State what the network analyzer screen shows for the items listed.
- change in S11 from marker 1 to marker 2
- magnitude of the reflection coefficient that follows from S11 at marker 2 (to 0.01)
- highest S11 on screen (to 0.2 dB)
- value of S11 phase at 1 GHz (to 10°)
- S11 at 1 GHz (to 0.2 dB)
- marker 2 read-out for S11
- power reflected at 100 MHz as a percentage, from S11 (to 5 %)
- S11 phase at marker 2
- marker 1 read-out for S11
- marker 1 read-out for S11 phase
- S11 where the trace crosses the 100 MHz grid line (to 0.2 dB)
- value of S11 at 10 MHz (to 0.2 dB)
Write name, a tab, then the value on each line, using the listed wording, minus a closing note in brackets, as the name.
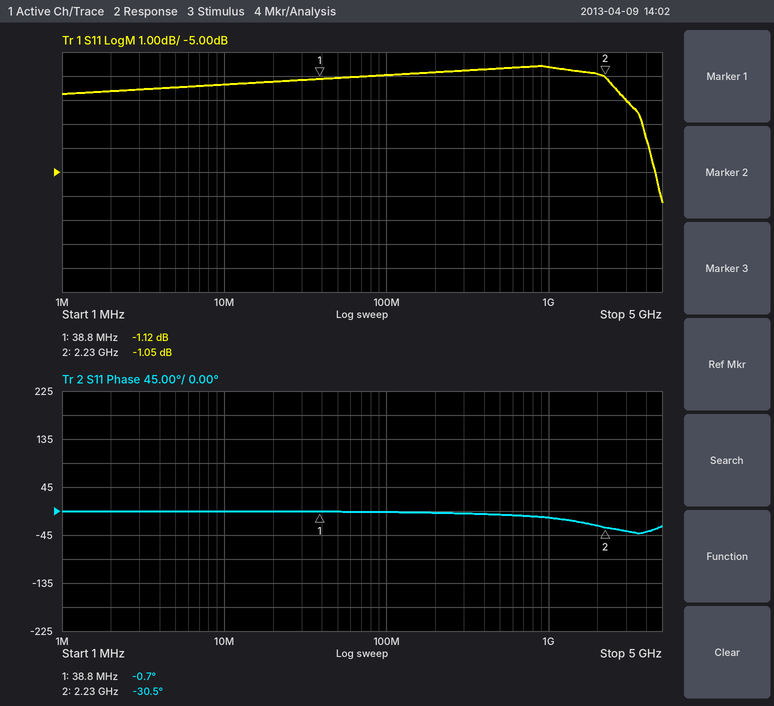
change in S11 from marker 1 to marker 2	0.07 dB
magnitude of the reflection coefficient that follows from S11 at marker 2	0.89
highest S11 on screen	-0.6 dB
value of S11 phase at 1 GHz	-10°
S11 at 1 GHz	-0.6 dB
marker 2 read-out for S11	-1.05 dB
power reflected at 100 MHz as a percentage, from S11	80 %
S11 phase at marker 2	-30.5°
marker 1 read-out for S11	-1.12 dB
marker 1 read-out for S11 phase	-0.7°
S11 where the trace crosses the 100 MHz grid line	-1.0 dB
value of S11 at 10 MHz	-1.4 dB
